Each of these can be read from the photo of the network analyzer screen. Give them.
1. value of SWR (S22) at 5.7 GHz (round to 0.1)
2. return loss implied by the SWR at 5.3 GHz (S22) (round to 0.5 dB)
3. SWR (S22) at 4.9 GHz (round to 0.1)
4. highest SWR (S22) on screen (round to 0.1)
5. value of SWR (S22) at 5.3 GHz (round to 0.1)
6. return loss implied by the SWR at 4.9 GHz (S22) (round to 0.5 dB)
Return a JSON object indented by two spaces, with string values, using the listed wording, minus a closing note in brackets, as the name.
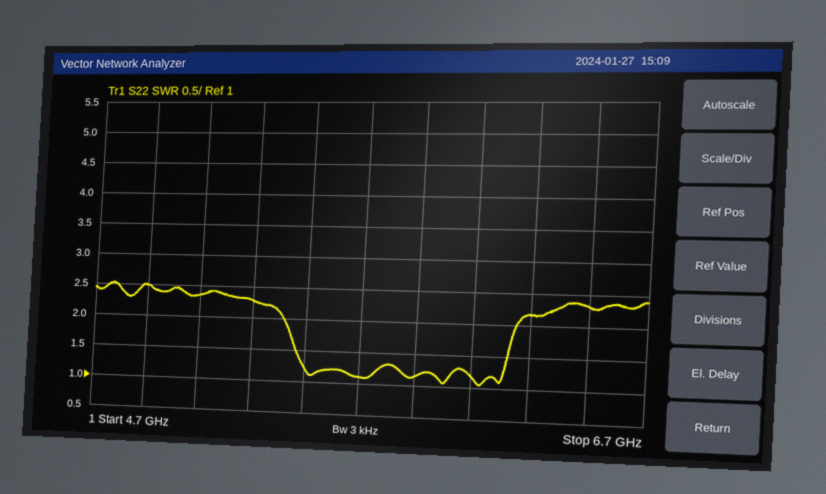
{
  "value of SWR (S22) at 5.7 GHz": "1.1",
  "return loss implied by the SWR at 5.3 GHz (S22)": "8.0 dB",
  "SWR (S22) at 4.9 GHz": "2.5",
  "highest SWR (S22) on screen": "2.5",
  "value of SWR (S22) at 5.3 GHz": "2.3",
  "return loss implied by the SWR at 4.9 GHz (S22)": "7.5 dB"
}
